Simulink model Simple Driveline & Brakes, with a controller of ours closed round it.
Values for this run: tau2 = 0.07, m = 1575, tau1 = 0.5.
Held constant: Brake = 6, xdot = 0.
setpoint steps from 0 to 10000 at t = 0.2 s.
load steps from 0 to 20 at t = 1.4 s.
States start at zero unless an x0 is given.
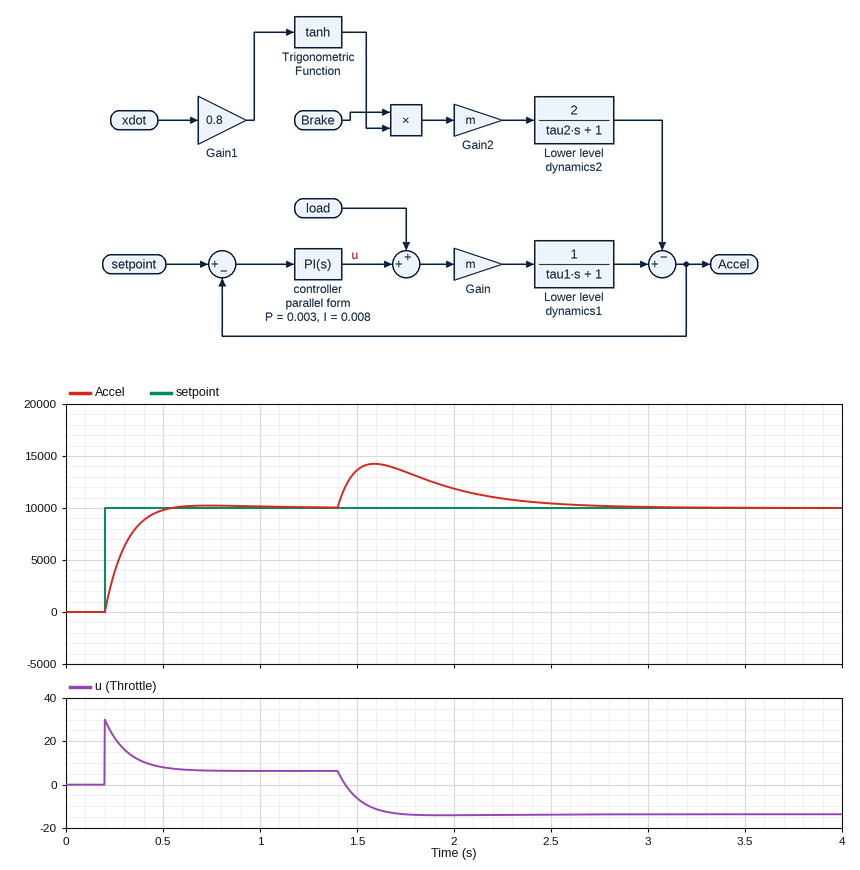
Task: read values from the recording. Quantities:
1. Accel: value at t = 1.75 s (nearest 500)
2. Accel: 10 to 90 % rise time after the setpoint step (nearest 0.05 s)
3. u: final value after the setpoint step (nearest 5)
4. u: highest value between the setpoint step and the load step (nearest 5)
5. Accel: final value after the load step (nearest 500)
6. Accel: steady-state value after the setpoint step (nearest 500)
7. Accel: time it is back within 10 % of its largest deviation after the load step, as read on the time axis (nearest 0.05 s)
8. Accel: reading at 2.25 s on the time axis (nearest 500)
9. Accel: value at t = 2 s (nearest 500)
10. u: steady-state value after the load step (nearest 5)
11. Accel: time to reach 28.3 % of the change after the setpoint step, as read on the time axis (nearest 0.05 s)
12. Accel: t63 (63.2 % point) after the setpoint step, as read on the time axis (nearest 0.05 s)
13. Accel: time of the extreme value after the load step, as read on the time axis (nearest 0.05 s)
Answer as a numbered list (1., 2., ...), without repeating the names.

1. 13500
2. 0.20 s
3. 5
4. 30
5. 10000
6. 10000
7. 2.50 s
8. 11000
9. 12000
10. -15
11. 0.25 s
12. 0.30 s
13. 1.60 s
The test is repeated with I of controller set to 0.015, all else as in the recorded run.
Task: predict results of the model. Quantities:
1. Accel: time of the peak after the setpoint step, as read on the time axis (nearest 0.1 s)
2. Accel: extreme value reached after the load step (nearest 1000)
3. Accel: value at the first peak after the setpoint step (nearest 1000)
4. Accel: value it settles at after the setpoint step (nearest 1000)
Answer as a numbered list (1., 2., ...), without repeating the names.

1. 0.6 s
2. 14000
3. 11000
4. 10000
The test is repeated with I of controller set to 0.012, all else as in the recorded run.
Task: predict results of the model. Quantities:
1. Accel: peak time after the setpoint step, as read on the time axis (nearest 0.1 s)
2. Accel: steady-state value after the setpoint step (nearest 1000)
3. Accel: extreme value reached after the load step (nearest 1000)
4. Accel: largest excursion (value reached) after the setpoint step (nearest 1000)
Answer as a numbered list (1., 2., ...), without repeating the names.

1. 0.6 s
2. 10000
3. 14000
4. 11000
